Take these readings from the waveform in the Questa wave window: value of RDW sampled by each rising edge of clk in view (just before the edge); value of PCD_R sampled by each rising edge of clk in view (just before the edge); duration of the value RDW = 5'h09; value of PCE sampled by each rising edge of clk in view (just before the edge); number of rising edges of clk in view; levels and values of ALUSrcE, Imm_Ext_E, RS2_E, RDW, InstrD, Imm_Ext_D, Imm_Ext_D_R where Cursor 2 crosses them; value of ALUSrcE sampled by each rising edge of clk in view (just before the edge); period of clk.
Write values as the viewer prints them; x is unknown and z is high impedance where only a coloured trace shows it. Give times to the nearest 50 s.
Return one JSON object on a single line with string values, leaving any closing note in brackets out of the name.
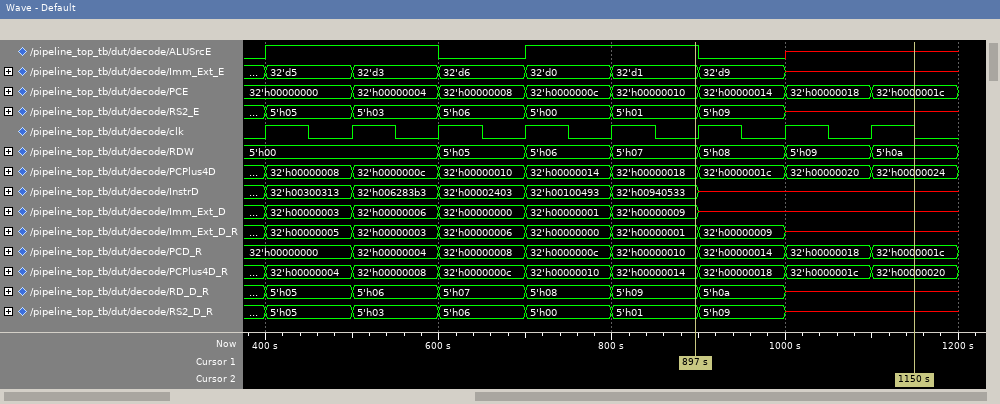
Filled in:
{"value of RDW sampled by each rising edge of clk in view": "5'h00, 5'h00, 5'h00, 5'h05, 5'h06, 5'h07, 5'h08, 5'h09", "value of PCD_R sampled by each rising edge of clk in view": "32'h00000000, 32'h00000000, 32'h00000004, 32'h00000008, 32'h0000000c, 32'h00000010, 32'h00000014, 32'h00000018", "duration of the value RDW = 5'h09": "100 s", "value of PCE sampled by each rising edge of clk in view": "32'h00000000, 32'h00000000, 32'h00000004, 32'h00000008, 32'h0000000c, 32'h00000010, 32'h00000014, 32'h00000018", "number of rising edges of clk in view": "8", "levels and values of ALUSrcE, Imm_Ext_E, RS2_E, RDW, InstrD, Imm_Ext_D, Imm_Ext_D_R where Cursor 2 crosses them": "ALUSrcE=x, Imm_Ext_E=x, RS2_E=x, RDW=5'h0a, InstrD=x, Imm_Ext_D=x, Imm_Ext_D_R=x", "value of ALUSrcE sampled by each rising edge of clk in view": "0 1 1 0 1 1 0 x", "period of clk": "100 s"}
